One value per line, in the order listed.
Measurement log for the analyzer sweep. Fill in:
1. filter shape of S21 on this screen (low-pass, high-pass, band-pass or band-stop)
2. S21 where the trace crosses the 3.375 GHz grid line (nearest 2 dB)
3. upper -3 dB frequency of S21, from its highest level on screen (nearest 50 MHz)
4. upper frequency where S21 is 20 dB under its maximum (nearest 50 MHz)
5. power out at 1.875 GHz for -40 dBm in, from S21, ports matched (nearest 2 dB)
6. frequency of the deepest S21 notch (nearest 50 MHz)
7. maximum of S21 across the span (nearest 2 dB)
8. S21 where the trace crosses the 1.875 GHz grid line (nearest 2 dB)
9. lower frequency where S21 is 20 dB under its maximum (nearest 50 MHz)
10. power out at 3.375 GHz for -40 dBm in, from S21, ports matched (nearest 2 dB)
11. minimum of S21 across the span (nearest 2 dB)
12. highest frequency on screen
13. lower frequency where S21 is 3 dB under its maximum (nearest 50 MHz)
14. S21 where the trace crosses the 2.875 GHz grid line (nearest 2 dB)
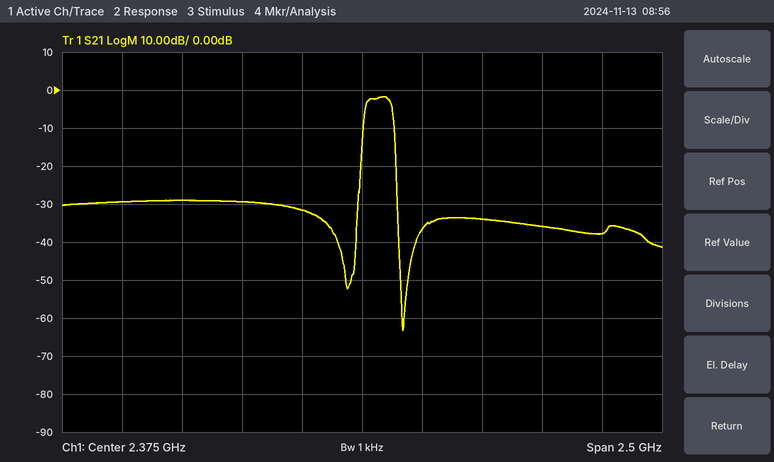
band-pass
-38 dB
2.50 GHz
2.50 GHz
-70 dBm
2.55 GHz
-2 dB
-30 dB
2.35 GHz
-78 dBm
-64 dB
3.625 GHz
2.40 GHz
-34 dB
